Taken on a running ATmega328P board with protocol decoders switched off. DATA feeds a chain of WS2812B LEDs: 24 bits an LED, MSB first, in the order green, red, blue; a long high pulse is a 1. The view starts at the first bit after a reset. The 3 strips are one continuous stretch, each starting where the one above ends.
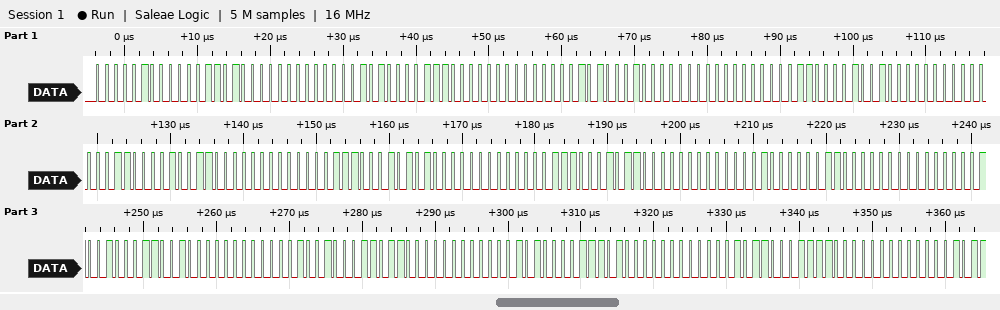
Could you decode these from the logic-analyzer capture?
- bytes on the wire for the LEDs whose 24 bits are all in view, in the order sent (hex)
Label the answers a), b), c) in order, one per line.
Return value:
a) 04 0D 00 05 0E 00 05 10 00 06 12 00 06 13 00 07 15 00 07 16 00 08 18 00 09 19 00 09 1B 00 0A 1D 00 0B 1E 00
